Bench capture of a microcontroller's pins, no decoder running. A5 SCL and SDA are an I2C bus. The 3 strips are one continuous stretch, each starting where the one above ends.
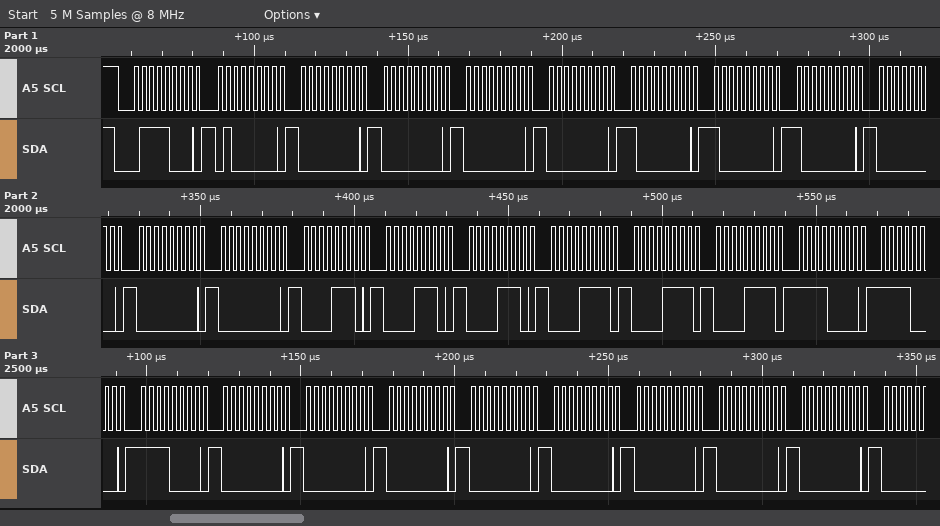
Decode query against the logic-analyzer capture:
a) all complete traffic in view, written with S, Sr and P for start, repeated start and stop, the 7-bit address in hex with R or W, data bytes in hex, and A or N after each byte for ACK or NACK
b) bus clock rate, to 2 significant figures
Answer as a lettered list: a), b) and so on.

a) S 3CW A 40 A 00 A 00 A 00 A 00 A 80 A 80 A 80 A 00 A 00 A 00 A 0E A 0E A 0E A 0F A 0F A 0F A F0 A F0 A F0 A 00 A 00 A 00 A 00 A 00 A 00 A 00 A 00 A
b) 400 kHz
